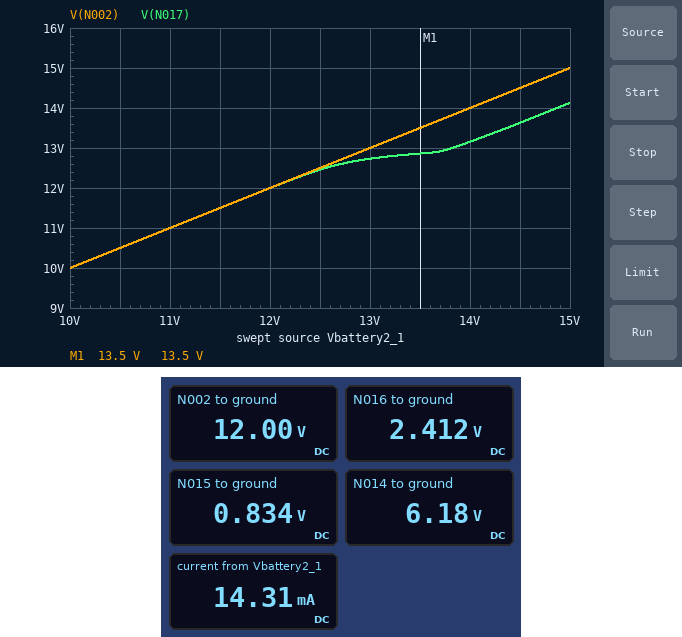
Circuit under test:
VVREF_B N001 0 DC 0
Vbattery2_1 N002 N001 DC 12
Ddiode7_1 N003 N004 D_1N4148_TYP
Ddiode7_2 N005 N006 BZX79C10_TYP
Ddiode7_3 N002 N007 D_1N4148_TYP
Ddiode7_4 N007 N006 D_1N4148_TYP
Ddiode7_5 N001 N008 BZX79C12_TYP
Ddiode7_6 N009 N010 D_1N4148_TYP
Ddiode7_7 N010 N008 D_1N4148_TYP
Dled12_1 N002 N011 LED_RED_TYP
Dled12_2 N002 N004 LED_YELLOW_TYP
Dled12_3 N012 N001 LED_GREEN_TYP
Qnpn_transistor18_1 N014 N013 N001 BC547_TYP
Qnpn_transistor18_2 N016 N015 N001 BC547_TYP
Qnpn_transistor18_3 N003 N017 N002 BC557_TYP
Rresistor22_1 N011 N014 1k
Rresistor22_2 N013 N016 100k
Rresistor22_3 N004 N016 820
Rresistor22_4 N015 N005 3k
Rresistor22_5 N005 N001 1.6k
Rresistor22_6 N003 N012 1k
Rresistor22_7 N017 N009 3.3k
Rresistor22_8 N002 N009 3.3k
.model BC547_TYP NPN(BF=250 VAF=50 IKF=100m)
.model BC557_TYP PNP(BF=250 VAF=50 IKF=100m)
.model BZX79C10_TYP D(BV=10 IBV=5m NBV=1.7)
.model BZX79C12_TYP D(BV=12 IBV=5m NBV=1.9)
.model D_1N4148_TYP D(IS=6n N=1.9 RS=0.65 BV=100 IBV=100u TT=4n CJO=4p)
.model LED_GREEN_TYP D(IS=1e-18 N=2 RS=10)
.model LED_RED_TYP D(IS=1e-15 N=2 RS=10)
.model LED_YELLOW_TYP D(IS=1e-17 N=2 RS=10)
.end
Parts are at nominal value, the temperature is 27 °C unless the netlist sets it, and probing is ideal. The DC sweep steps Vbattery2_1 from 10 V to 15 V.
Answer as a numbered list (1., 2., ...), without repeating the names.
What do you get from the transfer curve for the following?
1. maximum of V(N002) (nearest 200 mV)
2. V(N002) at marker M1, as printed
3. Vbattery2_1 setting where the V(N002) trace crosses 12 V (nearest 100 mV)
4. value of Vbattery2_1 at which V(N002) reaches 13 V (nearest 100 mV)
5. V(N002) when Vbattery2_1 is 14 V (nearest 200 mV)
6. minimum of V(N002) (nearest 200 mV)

1. 15.0 V
2. 13.5 V
3. 12.0 V
4. 13.0 V
5. 14.0 V
6. 10.0 V
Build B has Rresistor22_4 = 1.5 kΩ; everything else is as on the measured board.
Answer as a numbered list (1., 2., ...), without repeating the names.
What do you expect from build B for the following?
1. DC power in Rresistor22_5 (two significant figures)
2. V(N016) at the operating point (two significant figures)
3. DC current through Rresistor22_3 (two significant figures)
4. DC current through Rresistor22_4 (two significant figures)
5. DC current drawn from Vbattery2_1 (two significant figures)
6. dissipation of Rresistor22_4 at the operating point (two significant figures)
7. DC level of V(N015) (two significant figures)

1. 560 µW
2. 180 mV
3. 12 mA
4. 70 µA
5. 13 mA
6. 7.3 µW
7. 840 mV
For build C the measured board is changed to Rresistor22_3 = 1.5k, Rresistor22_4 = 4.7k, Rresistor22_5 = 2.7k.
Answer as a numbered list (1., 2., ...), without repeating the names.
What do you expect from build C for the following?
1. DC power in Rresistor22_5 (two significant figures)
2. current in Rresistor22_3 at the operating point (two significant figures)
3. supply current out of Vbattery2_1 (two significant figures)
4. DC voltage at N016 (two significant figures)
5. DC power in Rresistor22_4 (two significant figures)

1. 380 µW
2. 6.7 mA
3. 7.1 mA
4. 170 mV
5. 7.5 µW
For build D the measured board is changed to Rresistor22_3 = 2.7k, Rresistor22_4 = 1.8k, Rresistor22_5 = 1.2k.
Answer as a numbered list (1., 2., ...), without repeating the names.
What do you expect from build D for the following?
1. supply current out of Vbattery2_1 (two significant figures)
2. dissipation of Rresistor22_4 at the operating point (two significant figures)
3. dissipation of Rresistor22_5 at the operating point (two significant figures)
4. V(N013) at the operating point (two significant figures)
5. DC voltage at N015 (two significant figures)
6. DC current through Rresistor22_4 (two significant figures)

1. 4.6 mA
2. 6.2 µW
3. 700 µW
4. 120 mV
5. 810 mV
6. 59 µA
